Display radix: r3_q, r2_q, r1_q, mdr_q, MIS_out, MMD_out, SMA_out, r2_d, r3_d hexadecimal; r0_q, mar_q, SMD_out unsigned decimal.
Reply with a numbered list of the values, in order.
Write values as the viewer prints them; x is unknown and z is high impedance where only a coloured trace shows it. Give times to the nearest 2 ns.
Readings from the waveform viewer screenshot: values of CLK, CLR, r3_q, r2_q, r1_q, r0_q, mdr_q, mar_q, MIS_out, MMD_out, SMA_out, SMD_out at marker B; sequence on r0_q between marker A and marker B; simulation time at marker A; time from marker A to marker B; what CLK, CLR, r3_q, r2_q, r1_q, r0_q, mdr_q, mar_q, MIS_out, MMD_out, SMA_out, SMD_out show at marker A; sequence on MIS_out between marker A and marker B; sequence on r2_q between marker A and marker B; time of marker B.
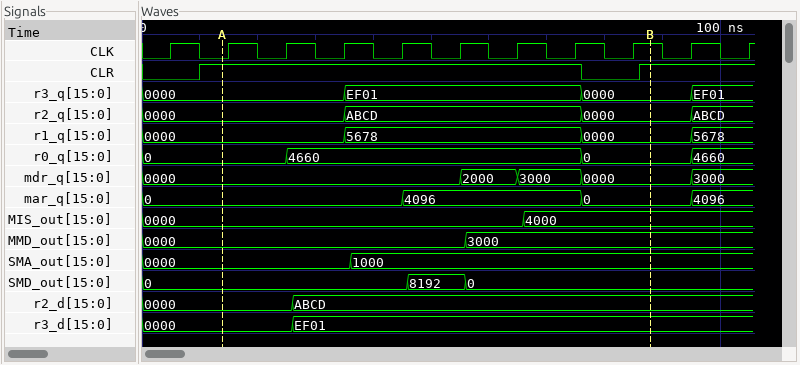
1. CLK=1, CLR=1, r3_q=0000, r2_q=0000, r1_q=0000, r0_q=0, mdr_q=0000, mar_q=0, MIS_out=4000, MMD_out=3000, SMA_out=1000, SMD_out=0
2. 0, 4660, 0
3. 14 ns
4. 74 ns
5. CLK=0, CLR=1, r3_q=0000, r2_q=0000, r1_q=0000, r0_q=0, mdr_q=0000, mar_q=0, MIS_out=0000, MMD_out=0000, SMA_out=0000, SMD_out=0
6. 0000, 4000
7. 0000, ABCD, 0000
8. 88 ns
